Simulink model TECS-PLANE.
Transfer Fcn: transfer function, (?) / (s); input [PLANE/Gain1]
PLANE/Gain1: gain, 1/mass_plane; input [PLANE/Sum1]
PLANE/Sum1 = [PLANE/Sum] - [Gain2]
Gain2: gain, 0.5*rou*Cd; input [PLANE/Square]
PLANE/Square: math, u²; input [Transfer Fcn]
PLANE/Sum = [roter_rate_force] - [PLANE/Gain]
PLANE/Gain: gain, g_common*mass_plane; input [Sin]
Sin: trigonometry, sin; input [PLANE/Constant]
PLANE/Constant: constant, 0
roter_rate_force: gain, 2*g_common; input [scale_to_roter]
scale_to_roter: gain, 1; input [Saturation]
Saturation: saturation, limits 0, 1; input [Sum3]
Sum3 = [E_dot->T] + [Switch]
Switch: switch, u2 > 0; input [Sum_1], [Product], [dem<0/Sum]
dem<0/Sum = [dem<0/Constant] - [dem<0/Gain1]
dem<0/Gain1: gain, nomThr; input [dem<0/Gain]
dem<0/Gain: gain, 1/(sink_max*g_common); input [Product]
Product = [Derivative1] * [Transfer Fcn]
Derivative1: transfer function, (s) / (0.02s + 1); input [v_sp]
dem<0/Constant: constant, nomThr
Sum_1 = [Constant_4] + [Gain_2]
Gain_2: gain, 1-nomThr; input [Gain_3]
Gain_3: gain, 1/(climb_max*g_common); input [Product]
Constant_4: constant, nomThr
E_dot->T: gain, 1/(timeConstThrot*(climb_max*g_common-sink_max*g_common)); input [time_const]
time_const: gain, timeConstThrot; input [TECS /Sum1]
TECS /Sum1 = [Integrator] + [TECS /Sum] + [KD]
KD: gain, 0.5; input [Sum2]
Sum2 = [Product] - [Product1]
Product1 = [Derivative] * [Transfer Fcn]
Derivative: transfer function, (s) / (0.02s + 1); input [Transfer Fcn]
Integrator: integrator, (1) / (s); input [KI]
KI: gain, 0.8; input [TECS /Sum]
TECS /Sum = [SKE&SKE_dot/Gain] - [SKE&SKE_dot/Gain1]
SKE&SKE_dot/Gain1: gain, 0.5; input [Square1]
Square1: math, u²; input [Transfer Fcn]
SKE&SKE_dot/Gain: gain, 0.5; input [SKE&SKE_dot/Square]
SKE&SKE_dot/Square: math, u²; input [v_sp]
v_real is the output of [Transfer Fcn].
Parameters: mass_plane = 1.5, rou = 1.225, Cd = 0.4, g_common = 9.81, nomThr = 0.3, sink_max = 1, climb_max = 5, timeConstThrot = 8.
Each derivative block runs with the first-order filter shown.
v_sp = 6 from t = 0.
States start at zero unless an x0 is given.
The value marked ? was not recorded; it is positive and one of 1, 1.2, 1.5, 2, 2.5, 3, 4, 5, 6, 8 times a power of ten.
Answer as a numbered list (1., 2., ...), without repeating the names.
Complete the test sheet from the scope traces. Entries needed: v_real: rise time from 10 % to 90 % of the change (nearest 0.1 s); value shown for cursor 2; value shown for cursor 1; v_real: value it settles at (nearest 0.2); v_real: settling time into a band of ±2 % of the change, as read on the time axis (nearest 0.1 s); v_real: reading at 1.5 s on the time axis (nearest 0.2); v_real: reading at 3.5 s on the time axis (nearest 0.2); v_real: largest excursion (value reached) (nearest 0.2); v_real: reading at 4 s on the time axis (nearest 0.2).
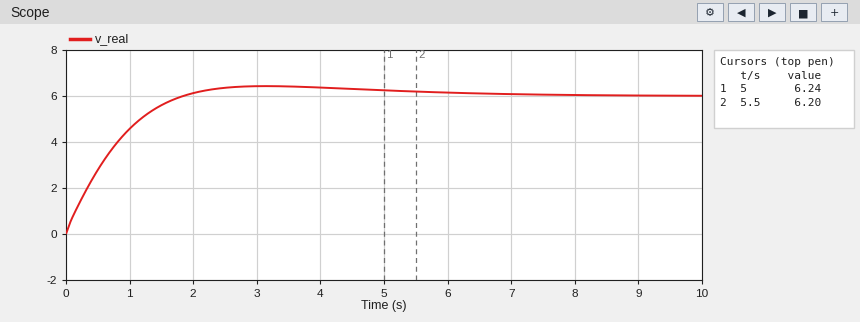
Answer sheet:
1. 1.3 s
2. 6.20
3. 6.24
4. 6.0
5. 6.4 s
6. 5.6
7. 6.4
8. 6.4
9. 6.4
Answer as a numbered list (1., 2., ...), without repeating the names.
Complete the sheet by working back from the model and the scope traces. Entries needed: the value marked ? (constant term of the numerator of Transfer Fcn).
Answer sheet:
1. 0.6
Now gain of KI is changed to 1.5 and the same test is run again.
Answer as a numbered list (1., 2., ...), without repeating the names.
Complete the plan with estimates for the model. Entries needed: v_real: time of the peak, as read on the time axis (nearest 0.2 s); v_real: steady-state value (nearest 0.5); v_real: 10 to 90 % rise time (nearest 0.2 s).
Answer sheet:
1. 2.4 s
2. 6.0
3. 1.0 s
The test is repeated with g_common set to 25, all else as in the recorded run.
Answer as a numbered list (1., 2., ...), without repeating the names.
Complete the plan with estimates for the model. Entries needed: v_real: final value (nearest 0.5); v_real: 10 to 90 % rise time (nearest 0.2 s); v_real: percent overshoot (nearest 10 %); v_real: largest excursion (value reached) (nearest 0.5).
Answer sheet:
1. 6.0
2. 0.8 s
3. 20 %
4. 7.0
